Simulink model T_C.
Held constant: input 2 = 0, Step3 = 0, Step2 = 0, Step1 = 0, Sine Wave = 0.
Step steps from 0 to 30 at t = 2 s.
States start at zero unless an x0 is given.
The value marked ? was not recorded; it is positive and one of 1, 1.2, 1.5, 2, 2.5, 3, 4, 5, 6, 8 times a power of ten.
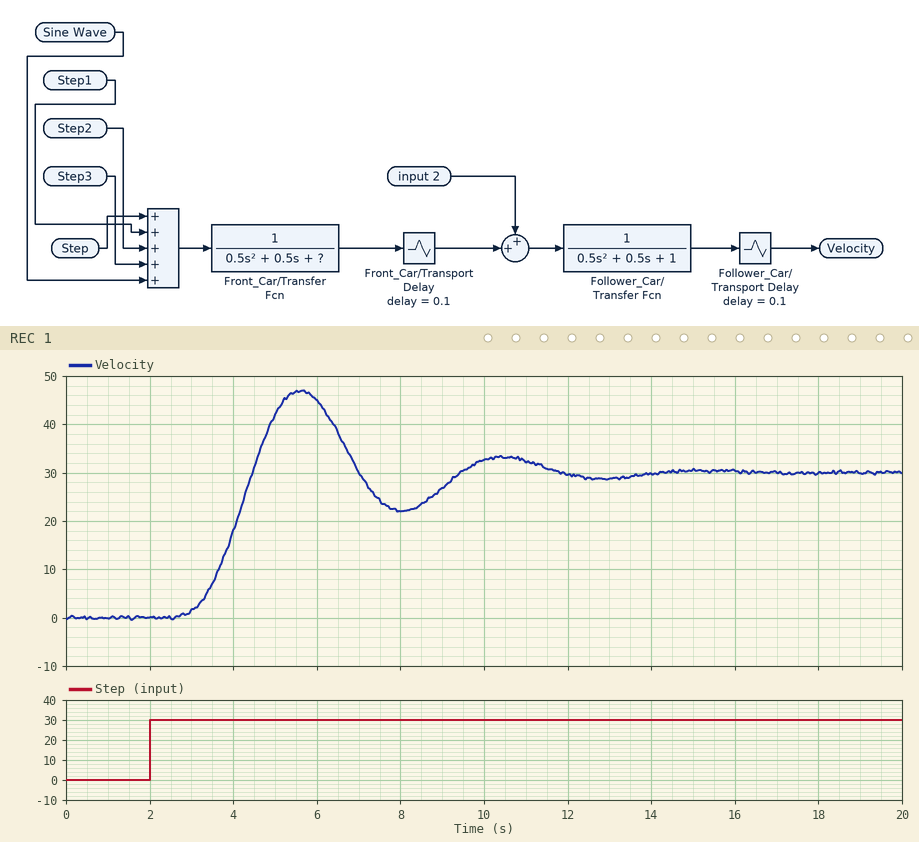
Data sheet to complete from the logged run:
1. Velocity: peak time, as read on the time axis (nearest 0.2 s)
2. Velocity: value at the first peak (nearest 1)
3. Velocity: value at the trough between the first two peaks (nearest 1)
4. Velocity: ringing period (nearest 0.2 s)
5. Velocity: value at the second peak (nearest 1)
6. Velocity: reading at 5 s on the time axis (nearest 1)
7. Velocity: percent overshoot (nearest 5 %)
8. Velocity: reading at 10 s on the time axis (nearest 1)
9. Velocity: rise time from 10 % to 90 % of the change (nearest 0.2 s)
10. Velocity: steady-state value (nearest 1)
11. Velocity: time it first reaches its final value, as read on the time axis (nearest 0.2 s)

5.6 s
47
22
4.8 s
33
42
55 %
33
1.2 s
30
4.4 s
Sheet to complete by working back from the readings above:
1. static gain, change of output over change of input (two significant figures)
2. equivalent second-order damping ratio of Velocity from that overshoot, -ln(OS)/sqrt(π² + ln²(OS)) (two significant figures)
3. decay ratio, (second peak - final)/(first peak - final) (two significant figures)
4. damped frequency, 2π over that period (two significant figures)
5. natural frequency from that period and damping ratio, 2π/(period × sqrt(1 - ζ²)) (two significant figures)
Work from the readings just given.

1.0
0.19
0.18
1.3 rad/s
1.3 rad/s
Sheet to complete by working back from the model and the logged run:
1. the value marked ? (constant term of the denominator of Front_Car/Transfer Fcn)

1
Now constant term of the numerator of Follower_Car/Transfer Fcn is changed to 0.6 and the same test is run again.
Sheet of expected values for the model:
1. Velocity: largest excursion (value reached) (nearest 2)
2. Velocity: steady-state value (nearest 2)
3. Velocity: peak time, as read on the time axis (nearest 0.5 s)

28
18
5.5 s
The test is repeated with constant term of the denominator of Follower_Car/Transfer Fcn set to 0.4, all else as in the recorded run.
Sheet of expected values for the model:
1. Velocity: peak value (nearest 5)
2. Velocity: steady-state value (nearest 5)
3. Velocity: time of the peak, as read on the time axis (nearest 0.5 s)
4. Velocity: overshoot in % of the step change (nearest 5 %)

95
75
6.5 s
25 %
